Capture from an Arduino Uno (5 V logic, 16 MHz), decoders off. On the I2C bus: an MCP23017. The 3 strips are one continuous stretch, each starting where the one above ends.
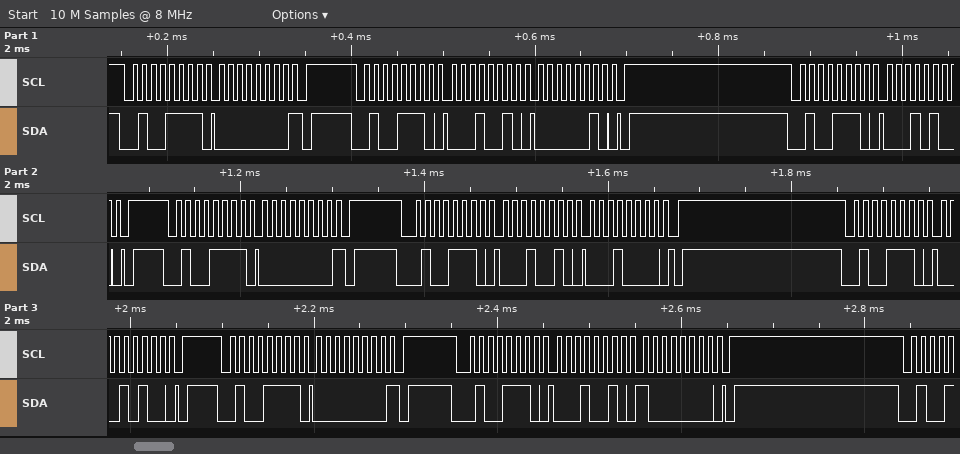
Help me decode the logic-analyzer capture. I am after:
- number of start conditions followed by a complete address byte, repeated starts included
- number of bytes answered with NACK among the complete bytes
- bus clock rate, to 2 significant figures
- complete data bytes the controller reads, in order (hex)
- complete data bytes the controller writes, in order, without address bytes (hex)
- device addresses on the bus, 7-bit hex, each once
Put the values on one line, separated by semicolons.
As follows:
8; 3; 100 kHz; 00 00 00; 12 02 14 12 10 14 12 80; 0x27
